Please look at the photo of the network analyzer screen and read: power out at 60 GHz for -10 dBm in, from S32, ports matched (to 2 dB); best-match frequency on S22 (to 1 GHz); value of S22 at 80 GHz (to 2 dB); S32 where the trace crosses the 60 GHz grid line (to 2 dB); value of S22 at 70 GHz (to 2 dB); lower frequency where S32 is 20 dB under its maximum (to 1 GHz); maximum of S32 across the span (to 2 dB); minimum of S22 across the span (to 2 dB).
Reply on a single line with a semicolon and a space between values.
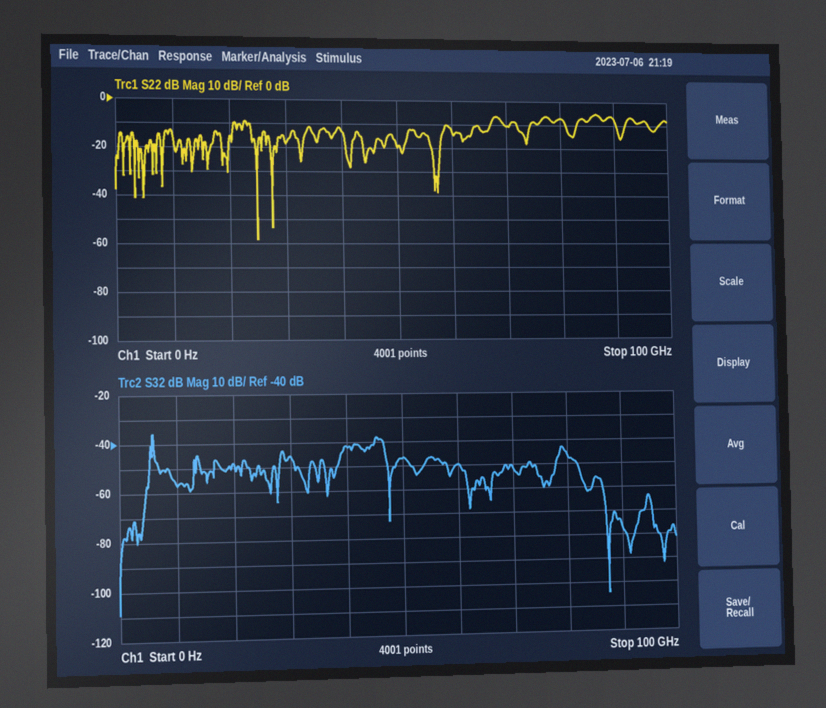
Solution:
-60 dBm; 25 GHz; -8 dB; -50 dB; -10 dB; 5 GHz; -36 dB; -58 dB
